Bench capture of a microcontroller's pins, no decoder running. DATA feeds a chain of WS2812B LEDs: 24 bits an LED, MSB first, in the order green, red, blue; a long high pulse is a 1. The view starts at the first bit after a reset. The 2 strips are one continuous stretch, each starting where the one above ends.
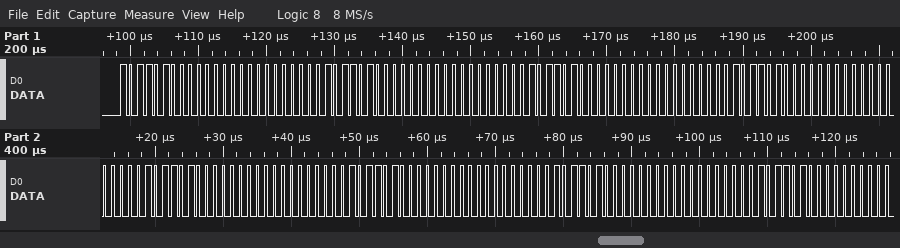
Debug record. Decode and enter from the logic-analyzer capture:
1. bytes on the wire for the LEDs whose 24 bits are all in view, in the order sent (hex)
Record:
B4 00 00 B4 00 00 B4 00 00 B4 00 00 B4 00 00 B4 00 00 B4 00 00
